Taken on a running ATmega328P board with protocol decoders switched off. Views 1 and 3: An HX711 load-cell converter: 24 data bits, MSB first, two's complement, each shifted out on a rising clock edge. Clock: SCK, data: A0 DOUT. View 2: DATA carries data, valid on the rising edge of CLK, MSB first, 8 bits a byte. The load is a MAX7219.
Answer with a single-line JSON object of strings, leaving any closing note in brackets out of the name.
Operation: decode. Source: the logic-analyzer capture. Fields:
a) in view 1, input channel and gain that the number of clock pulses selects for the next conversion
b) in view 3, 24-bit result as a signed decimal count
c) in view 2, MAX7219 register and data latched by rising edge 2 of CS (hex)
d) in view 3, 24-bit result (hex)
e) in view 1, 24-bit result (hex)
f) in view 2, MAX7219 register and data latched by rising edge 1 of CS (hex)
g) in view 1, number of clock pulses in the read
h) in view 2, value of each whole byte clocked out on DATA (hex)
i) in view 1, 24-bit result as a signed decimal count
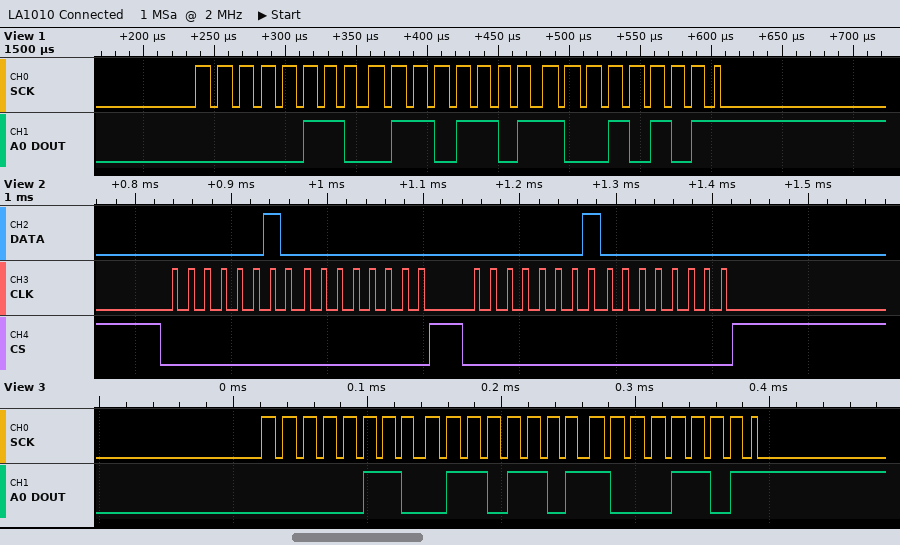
{"in view 1, input channel and gain that the number of clock pulses selects for the next conversion": "channel A, gain 128", "in view 3, 24-bit result as a signed decimal count": "421261", "in view 2, MAX7219 register and data latched by rising edge 2 of CS": "register 0x1, data 0x00", "in view 3, 24-bit result": "0x066D8D", "in view 1, 24-bit result": "0x066D95", "in view 2, MAX7219 register and data latched by rising edge 1 of CS": "register 0x2, data 0x00", "in view 1, number of clock pulses in the read": "25", "in view 2, value of each whole byte clocked out on DATA": "0x02 0x00 0x01 0x00", "in view 1, 24-bit result as a signed decimal count": "421269"}
